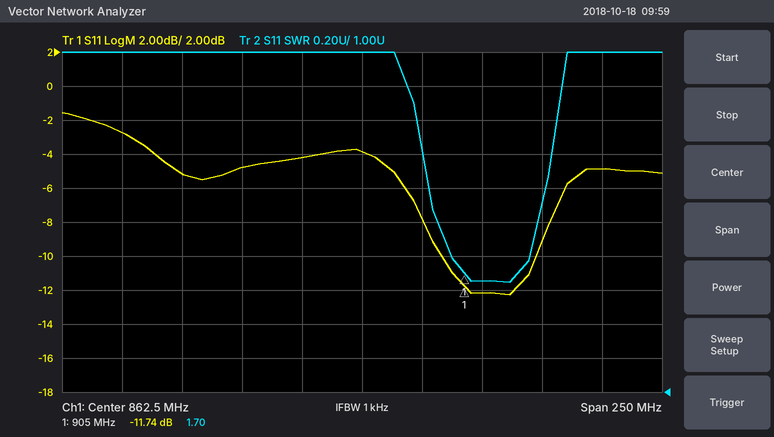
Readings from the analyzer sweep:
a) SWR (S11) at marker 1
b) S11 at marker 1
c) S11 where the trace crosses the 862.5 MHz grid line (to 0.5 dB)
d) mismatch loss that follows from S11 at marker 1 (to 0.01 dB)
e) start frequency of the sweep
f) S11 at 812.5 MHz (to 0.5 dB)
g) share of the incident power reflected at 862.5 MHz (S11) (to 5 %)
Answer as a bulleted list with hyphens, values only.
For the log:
- 1.70
- -11.74 dB
- -4.0 dB
- 0.30 dB
- 737.5 MHz
- -5.0 dB
- 40 %
